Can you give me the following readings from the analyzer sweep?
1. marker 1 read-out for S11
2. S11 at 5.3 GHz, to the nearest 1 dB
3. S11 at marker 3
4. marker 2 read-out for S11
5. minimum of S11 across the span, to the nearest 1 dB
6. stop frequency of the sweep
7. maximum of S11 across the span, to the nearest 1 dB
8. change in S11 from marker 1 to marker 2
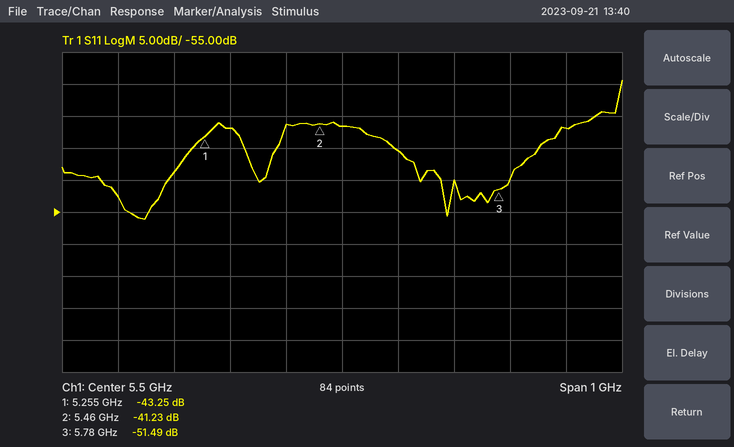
-43.25 dB
-42 dB
-51.49 dB
-41.23 dB
-56 dB
6 GHz
-34 dB
2.02 dB
